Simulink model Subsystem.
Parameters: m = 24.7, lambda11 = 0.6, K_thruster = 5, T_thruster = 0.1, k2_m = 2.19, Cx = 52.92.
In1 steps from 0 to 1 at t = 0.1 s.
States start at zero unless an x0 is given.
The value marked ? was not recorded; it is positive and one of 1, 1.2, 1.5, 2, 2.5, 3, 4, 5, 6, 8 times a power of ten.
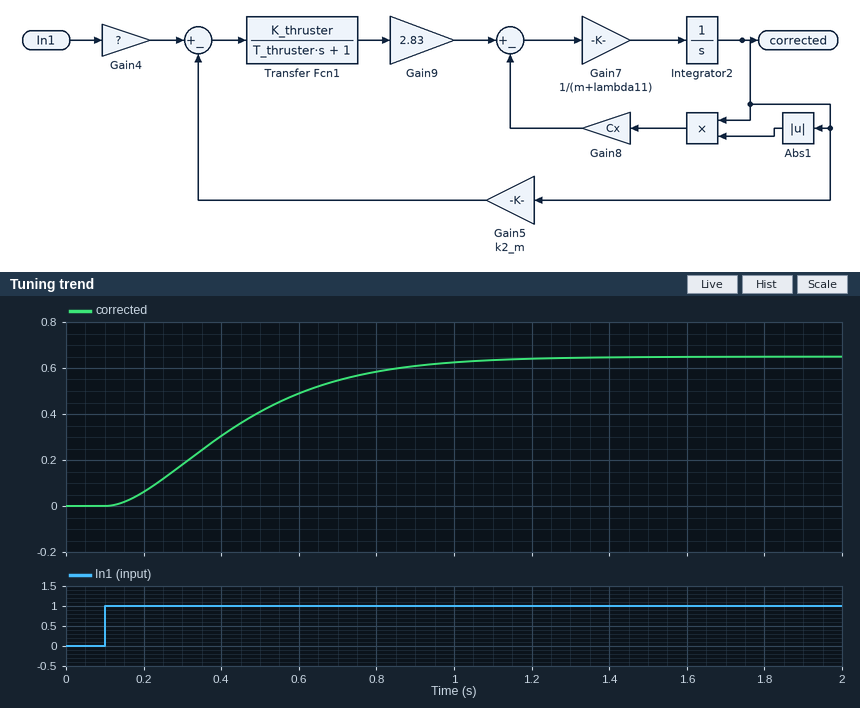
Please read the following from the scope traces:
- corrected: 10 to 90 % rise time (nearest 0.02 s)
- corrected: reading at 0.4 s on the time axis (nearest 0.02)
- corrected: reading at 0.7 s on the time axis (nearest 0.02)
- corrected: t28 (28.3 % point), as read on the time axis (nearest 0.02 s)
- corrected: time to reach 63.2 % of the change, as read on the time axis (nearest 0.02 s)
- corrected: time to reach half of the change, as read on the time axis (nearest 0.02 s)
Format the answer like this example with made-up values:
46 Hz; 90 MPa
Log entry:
0.60 s; 0.30; 0.54; 0.30 s; 0.50 s; 0.42 s
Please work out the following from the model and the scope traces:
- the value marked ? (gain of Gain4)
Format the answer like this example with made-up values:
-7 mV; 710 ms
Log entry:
3
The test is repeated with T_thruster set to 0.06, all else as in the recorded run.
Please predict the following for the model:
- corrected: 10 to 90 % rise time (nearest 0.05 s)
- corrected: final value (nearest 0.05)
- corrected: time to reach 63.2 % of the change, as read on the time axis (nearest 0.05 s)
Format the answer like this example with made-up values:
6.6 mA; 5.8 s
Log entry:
0.60 s; 0.65; 0.45 s
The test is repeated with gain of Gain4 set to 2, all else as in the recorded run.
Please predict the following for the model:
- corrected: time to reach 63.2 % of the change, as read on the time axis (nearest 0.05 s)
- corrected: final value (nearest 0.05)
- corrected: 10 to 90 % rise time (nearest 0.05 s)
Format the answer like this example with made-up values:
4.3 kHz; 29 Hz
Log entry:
0.55 s; 0.50; 0.70 s
